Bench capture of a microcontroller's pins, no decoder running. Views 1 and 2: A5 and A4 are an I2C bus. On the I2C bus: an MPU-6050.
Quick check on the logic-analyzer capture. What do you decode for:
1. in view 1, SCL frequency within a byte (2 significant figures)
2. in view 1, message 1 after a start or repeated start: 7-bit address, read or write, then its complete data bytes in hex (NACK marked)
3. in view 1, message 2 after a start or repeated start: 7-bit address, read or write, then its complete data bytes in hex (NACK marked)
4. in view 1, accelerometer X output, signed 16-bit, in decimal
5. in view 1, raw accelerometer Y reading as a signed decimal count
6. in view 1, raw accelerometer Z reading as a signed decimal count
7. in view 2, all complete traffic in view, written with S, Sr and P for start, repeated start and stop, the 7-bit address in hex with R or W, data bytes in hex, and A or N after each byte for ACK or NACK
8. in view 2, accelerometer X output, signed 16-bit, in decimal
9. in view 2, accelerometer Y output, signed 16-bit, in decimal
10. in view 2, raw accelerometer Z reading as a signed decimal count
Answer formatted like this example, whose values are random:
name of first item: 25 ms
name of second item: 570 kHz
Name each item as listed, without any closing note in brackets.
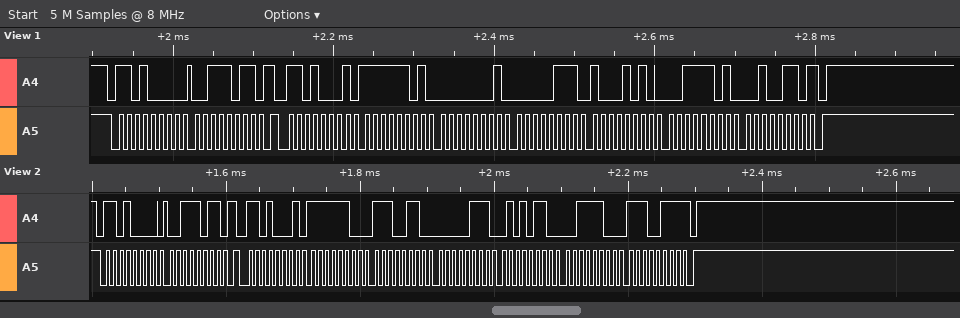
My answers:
in view 1, SCL frequency within a byte: 100 kHz
in view 1, message 1 after a start or repeated start: 7-bit address, read or write, then its complete data bytes in hex: 0x68 write: 3B
in view 1, message 2 after a start or repeated start: 7-bit address, read or write, then its complete data bytes in hex: 0x68 read: FD 01 07 8A 3D 26 NACK
in view 1, accelerometer X output, signed 16-bit, in decimal: -767
in view 1, raw accelerometer Y reading as a signed decimal count: 1930
in view 1, raw accelerometer Z reading as a signed decimal count: 15654
in view 2, all complete traffic in view, written with S, Sr and P for start, repeated start and stop, the 7-bit address in hex with R or W, data bytes in hex, and A or N after each byte for ACK or NACK: S 68W A 3B A Sr 68R A FC A E6 A 07 A 56 A 3C A E7 N P
in view 2, accelerometer X output, signed 16-bit, in decimal: -794
in view 2, accelerometer Y output, signed 16-bit, in decimal: 1878
in view 2, raw accelerometer Z reading as a signed decimal count: 15591
